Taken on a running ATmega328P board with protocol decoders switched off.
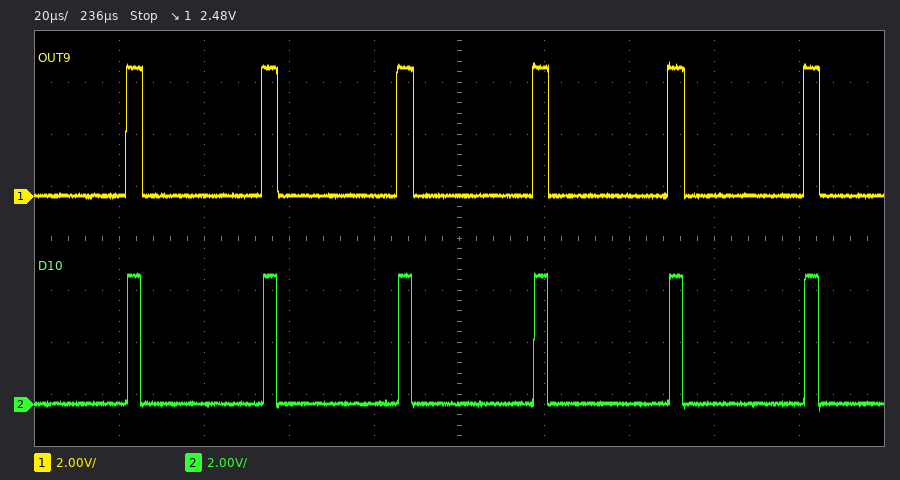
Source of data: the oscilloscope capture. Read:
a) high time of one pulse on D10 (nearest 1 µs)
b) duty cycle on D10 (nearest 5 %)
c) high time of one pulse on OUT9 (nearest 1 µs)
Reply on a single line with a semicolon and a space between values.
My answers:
3 µs; 10 %; 4 µs
